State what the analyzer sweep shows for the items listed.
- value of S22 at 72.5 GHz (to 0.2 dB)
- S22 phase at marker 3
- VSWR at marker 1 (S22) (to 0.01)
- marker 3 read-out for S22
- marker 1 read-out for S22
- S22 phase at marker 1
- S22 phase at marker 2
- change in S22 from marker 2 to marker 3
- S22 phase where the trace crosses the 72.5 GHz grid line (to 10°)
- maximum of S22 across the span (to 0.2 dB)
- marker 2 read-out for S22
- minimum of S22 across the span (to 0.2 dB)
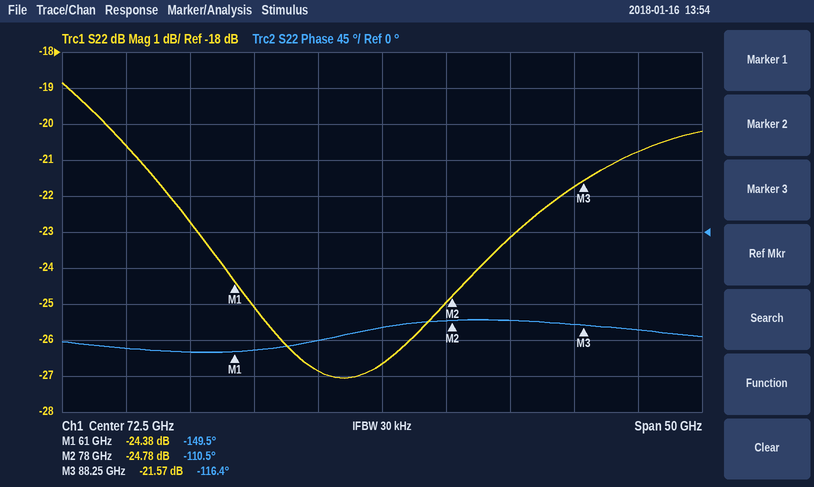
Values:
-26.6 dB
-116.4°
1.13
-21.57 dB
-24.38 dB
-149.5°
-110.5°
3.21 dB
-120°
-18.8 dB
-24.78 dB
-27.0 dB
